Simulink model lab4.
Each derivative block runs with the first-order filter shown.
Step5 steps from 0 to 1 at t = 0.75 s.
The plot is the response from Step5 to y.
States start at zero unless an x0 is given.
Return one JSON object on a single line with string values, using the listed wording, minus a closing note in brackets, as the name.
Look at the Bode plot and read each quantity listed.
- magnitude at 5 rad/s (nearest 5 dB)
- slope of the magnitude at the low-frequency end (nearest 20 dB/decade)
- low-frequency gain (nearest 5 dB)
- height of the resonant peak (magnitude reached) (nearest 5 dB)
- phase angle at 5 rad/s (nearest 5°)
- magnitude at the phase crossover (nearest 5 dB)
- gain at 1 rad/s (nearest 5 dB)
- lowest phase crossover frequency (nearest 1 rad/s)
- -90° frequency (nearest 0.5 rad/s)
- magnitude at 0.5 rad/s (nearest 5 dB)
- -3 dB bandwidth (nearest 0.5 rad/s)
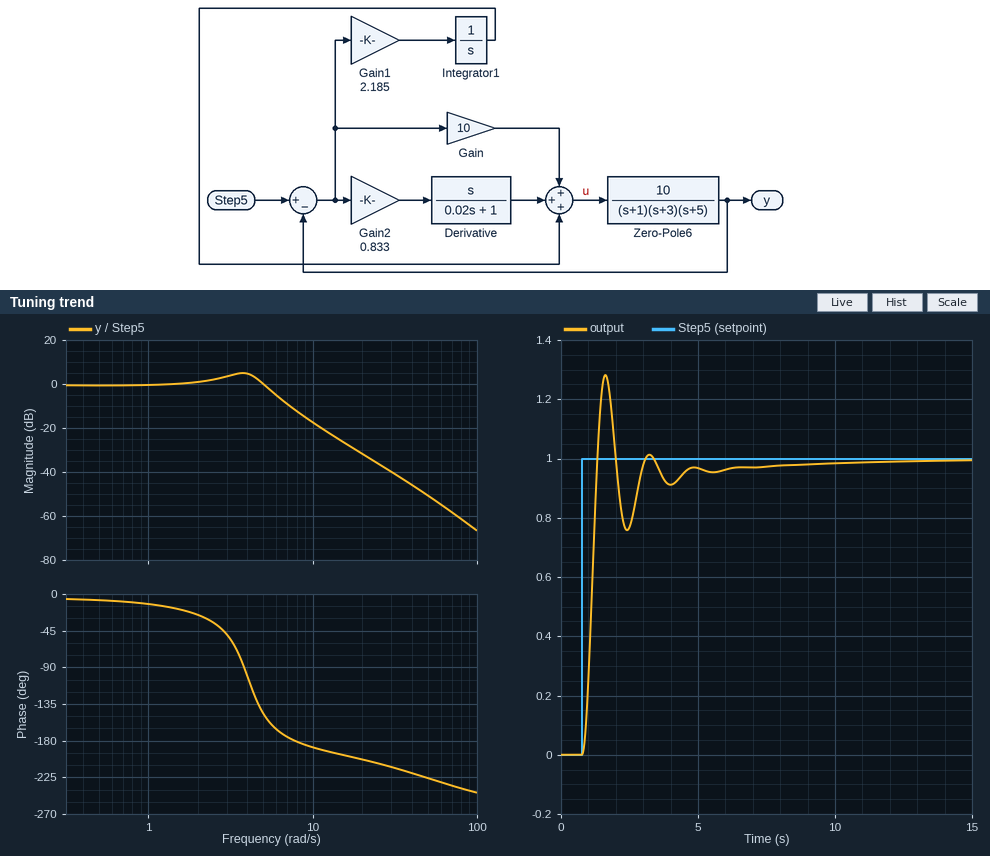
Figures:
{"magnitude at 5 rad/s": "0 dB", "slope of the magnitude at the low-frequency end": "0 dB/decade", "low-frequency gain": "0 dB", "height of the resonant peak (magnitude reached)": "5 dB", "phase angle at 5 rad/s": "-145°", "magnitude at the phase crossover": "-10 dB", "gain at 1 rad/s": "0 dB", "lowest phase crossover frequency": "8 rad/s", "-90° frequency": "4.0 rad/s", "magnitude at 0.5 rad/s": "0 dB", "-3 dB bandwidth": "5.5 rad/s"}
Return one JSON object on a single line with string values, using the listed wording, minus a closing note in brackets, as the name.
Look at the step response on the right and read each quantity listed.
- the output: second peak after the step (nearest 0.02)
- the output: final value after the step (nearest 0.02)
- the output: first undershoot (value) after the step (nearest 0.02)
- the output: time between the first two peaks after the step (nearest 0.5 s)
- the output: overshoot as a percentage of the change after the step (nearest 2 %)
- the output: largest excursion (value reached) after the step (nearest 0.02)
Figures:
{"the output: second peak after the step": "1.02", "the output: final value after the step": "1.00", "the output: first undershoot (value) after the step": "0.76", "the output: time between the first two peaks after the step": "1.5 s", "the output: overshoot as a percentage of the change after the step": "28 %", "the output: largest excursion (value reached) after the step": "1.28"}
